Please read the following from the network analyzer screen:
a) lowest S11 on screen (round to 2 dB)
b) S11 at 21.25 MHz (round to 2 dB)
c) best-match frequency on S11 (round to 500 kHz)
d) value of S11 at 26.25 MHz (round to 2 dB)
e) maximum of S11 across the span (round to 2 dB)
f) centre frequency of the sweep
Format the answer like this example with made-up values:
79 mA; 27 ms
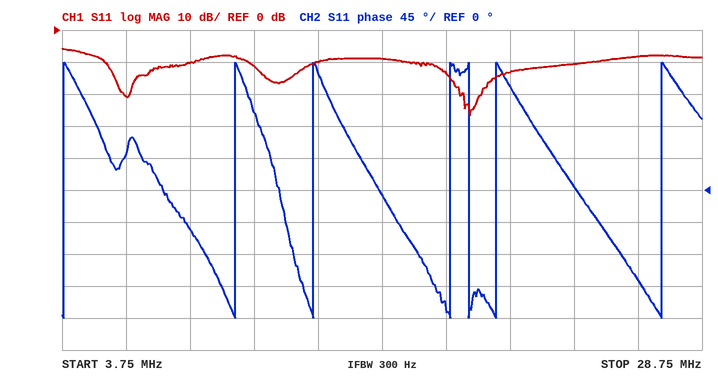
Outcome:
-26 dB; -14 dB; 19.5 MHz; -8 dB; -6 dB; 16.25 MHz
